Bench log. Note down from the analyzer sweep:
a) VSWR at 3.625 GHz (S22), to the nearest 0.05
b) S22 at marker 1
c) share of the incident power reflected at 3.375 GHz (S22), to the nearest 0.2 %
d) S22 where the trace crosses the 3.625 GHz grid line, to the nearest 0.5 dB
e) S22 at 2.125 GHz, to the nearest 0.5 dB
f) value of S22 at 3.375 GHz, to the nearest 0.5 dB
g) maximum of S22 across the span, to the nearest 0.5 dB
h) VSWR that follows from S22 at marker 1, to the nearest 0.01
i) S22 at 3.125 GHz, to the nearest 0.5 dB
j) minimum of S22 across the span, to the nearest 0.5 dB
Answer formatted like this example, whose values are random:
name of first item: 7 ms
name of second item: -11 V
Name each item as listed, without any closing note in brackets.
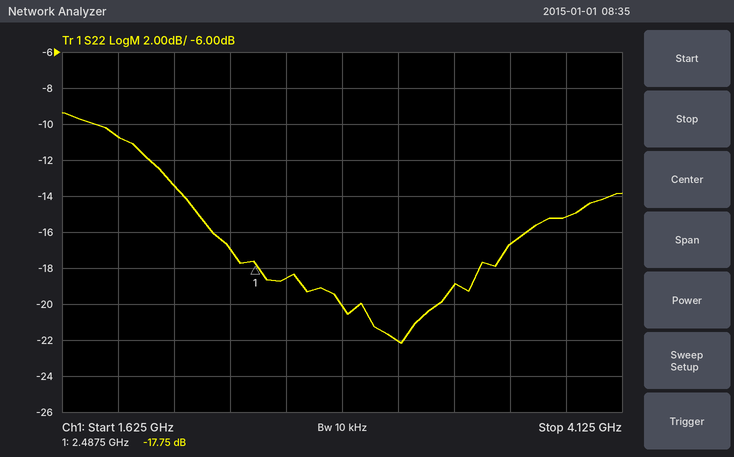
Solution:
VSWR at 3.625 GHz (S22), to the nearest 0.05: 1.35
S22 at marker 1: -17.75 dB
share of the incident power reflected at 3.375 GHz (S22), to the nearest 0.2 %: 1.2 %
S22 where the trace crosses the 3.625 GHz grid line, to the nearest 0.5 dB: -16.5 dB
S22 at 2.125 GHz, to the nearest 0.5 dB: -13.5 dB
value of S22 at 3.375 GHz, to the nearest 0.5 dB: -19.0 dB
maximum of S22 across the span, to the nearest 0.5 dB: -9.5 dB
VSWR that follows from S22 at marker 1, to the nearest 0.01: 1.30
S22 at 3.125 GHz, to the nearest 0.5 dB: -22.0 dB
minimum of S22 across the span, to the nearest 0.5 dB: -22.0 dB
